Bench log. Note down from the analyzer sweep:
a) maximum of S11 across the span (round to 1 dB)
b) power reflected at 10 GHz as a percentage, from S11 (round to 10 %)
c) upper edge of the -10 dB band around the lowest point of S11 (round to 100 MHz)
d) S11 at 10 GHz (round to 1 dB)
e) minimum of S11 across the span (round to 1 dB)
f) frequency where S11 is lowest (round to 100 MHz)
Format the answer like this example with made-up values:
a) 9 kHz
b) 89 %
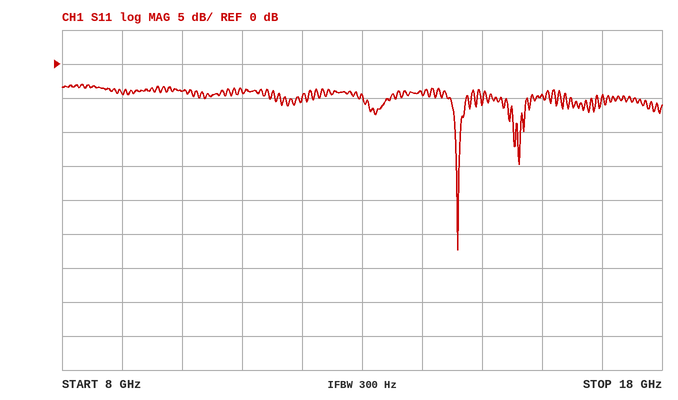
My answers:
a) -3 dB
b) 40 %
c) 14.6 GHz
d) -4 dB
e) -27 dB
f) 14.6 GHz
